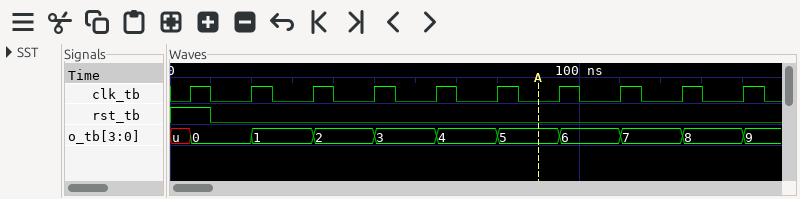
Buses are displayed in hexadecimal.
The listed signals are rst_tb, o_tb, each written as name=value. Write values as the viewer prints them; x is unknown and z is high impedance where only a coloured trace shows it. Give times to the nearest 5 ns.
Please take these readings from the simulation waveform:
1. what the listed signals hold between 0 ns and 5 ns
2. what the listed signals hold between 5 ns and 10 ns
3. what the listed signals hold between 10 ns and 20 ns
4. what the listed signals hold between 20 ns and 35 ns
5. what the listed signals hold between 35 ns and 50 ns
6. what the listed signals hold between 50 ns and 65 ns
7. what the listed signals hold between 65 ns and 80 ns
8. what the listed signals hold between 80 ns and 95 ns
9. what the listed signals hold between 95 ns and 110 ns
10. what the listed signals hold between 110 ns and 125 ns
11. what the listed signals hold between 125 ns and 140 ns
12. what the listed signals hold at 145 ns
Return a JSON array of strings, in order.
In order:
["rst_tb=1, o_tb=u", "rst_tb=1, o_tb=0", "rst_tb=0, o_tb=0", "rst_tb=0, o_tb=1", "rst_tb=0, o_tb=2", "rst_tb=0, o_tb=3", "rst_tb=0, o_tb=4", "rst_tb=0, o_tb=5", "rst_tb=0, o_tb=6", "rst_tb=0, o_tb=7", "rst_tb=0, o_tb=8", "rst_tb=0, o_tb=9"]
